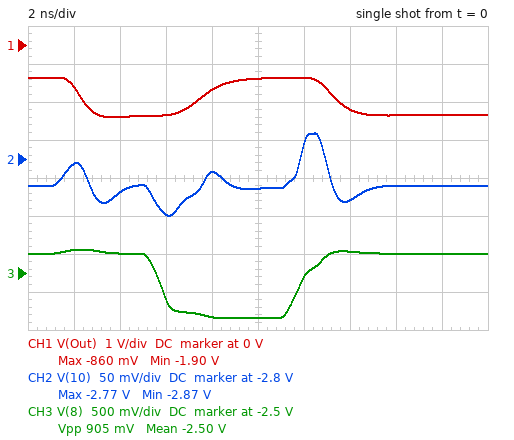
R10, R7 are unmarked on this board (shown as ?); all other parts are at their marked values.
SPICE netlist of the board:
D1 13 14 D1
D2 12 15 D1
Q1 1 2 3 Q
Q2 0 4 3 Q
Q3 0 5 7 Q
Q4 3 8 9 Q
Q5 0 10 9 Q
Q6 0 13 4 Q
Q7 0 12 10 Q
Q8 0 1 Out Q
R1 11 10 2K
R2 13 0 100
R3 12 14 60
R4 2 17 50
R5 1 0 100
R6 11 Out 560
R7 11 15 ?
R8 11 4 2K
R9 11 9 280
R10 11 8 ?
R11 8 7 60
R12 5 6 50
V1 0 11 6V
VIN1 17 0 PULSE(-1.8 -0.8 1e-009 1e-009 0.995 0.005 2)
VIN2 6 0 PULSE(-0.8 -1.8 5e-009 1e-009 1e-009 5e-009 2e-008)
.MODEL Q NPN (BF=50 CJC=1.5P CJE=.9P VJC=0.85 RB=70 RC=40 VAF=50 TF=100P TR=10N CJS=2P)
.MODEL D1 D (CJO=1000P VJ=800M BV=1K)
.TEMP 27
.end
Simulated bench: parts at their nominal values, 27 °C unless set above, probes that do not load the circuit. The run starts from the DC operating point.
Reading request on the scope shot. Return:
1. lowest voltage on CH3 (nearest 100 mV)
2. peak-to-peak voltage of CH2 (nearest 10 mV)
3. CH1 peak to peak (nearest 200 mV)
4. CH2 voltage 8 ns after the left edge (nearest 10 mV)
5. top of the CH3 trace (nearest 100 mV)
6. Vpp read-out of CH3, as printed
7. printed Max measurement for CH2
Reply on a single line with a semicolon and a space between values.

-3.1 V; 110 mV; 1.0 V; -2.82 V; -2.2 V; 905 mV; -2.77 V
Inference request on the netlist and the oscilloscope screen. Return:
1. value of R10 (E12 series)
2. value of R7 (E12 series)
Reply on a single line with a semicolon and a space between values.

390 Ω; 390 Ω
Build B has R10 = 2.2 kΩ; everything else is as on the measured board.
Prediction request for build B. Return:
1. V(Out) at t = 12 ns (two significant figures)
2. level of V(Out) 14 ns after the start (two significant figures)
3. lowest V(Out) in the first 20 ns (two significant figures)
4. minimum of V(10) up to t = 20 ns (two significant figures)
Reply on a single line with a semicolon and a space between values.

-1.9 V; -2.0 V; -2.1 V; -2.9 V
